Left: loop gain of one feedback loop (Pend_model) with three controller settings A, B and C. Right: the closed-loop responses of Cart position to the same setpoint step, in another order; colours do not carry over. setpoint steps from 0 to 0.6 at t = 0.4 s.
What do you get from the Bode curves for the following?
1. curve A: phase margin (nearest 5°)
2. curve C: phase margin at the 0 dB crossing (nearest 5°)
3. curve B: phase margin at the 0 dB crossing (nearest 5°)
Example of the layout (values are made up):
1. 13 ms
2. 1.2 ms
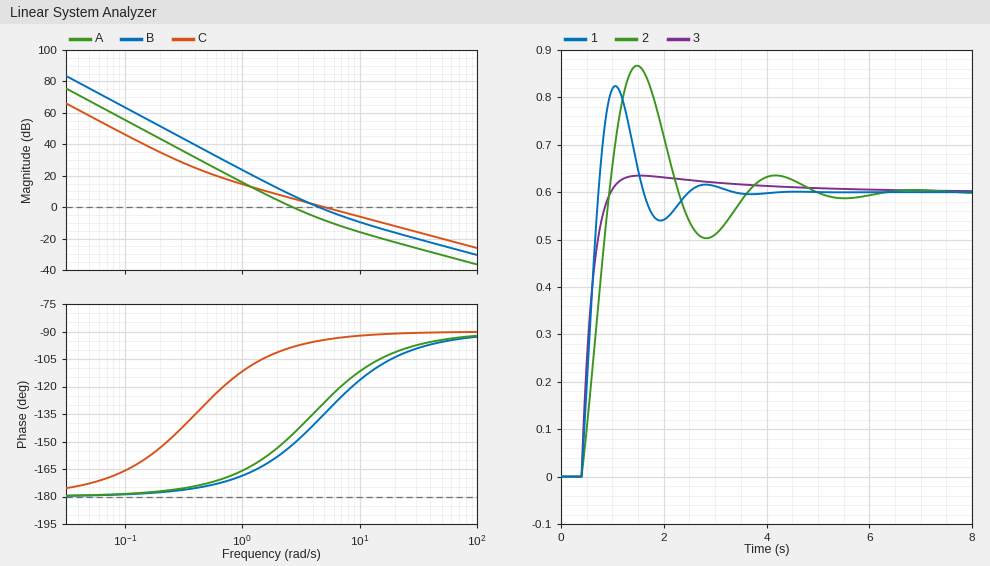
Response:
1. 35°
2. 85°
3. 40°
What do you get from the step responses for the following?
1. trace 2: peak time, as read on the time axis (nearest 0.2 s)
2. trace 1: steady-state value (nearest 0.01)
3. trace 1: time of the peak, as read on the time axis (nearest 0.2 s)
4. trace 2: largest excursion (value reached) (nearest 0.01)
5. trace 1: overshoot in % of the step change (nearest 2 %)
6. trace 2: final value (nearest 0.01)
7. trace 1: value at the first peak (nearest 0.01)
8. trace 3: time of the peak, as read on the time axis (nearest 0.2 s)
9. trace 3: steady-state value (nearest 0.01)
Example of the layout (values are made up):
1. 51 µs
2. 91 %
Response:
1. 1.4 s
2. 0.60
3. 1.0 s
4. 0.87
5. 38 %
6. 0.60
7. 0.82
8. 1.6 s
9. 0.60
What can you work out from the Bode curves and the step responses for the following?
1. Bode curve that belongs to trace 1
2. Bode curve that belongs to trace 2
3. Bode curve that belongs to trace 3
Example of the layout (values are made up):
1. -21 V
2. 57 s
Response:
1. B
2. A
3. C
